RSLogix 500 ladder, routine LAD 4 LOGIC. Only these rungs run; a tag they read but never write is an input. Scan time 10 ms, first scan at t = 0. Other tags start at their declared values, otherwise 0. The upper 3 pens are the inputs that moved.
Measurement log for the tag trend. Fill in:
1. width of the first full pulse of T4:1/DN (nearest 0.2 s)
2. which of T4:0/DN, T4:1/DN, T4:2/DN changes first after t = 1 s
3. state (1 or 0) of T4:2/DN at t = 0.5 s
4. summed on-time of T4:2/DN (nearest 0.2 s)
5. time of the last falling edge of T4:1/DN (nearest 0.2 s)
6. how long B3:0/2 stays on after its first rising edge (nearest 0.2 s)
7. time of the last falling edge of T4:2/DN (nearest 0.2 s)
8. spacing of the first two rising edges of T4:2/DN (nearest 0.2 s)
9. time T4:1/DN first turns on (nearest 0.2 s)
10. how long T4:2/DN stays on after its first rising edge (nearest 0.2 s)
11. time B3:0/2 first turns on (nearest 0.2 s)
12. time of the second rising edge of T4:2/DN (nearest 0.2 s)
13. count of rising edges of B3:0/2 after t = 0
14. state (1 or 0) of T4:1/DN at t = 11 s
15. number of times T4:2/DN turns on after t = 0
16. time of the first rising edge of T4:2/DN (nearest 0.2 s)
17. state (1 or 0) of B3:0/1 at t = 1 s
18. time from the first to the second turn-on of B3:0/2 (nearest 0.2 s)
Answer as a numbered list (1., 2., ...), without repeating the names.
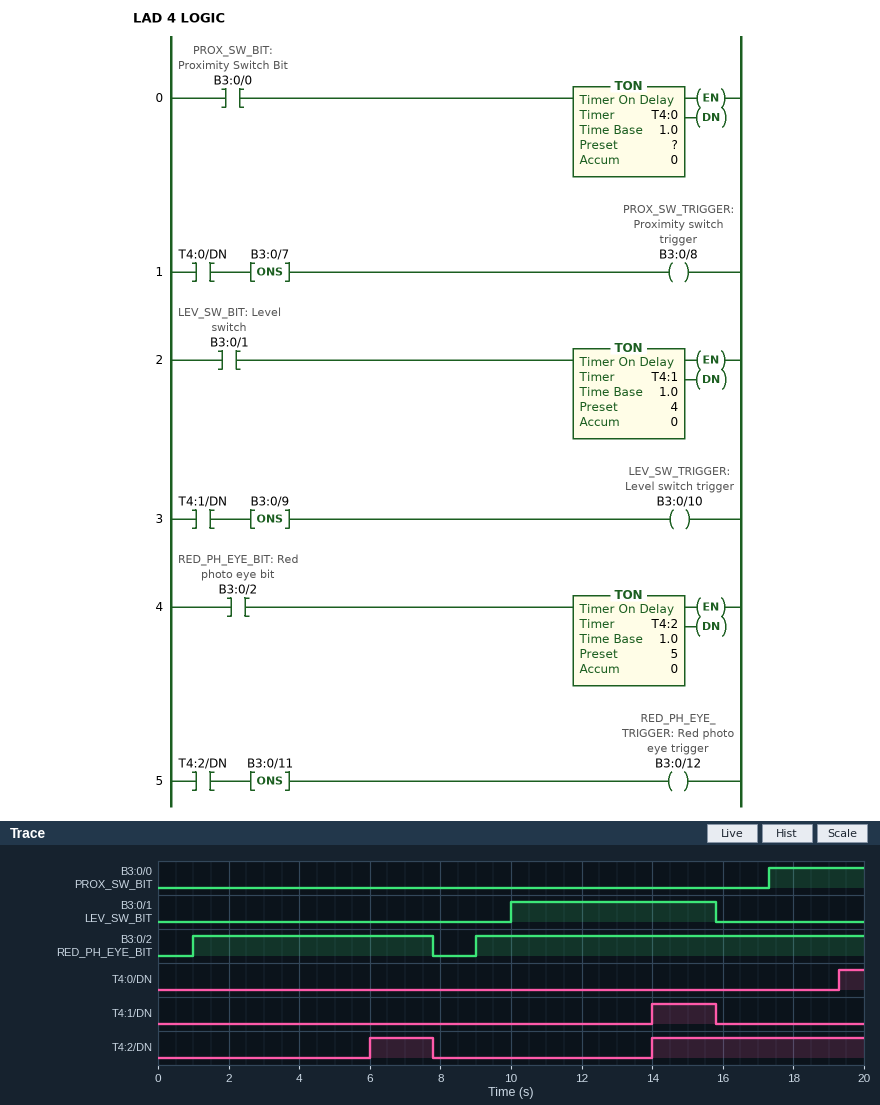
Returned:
1. 1.8 s
2. T4:2/DN
3. 0
4. 7.8 s
5. 15.8 s
6. 6.8 s
7. 7.8 s
8. 8.0 s
9. 14.0 s
10. 1.8 s
11. 1.0 s
12. 14.0 s
13. 2
14. 0
15. 2
16. 6.0 s
17. 0
18. 8.0 s
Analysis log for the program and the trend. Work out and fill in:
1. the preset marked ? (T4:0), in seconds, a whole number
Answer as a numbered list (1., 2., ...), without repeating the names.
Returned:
1. 2 s
